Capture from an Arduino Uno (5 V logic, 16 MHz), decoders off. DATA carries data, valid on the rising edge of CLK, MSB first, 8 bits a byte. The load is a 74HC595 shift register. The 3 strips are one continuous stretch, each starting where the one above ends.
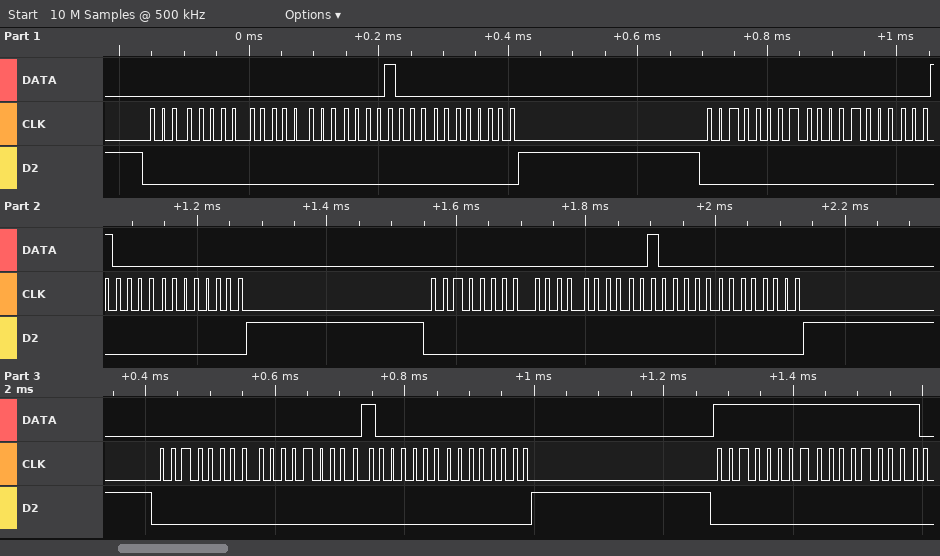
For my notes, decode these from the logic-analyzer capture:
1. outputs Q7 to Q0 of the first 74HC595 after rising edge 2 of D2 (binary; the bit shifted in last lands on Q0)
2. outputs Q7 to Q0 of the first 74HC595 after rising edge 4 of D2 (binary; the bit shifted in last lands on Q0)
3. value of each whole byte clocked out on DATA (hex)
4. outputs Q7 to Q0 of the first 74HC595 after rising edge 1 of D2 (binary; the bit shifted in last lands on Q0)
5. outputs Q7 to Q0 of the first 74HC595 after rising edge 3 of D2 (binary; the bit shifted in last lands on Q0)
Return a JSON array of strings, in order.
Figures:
["00000000", "00000000", "00 00 08 00 00 00 10 00 00 00 20 00 00 00 40 00 FF FF", "00000000", "00000000"]
